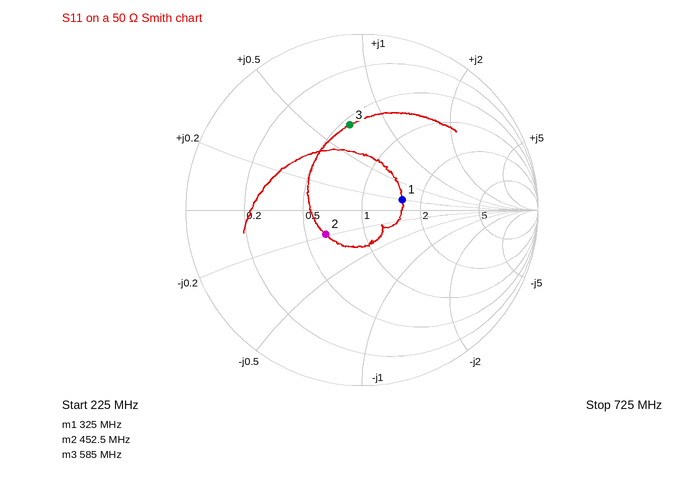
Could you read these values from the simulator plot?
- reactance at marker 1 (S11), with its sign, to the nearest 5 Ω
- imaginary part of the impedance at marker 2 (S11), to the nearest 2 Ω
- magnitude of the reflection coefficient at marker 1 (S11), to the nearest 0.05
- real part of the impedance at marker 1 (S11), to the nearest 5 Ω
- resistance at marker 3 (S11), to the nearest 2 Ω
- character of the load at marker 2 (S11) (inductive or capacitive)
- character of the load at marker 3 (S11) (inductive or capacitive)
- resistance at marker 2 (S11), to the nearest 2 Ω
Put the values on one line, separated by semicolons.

+10 Ω; -10 Ω; 0.25; 80 Ω; 28 Ω; capacitive; inductive; 32 Ω
